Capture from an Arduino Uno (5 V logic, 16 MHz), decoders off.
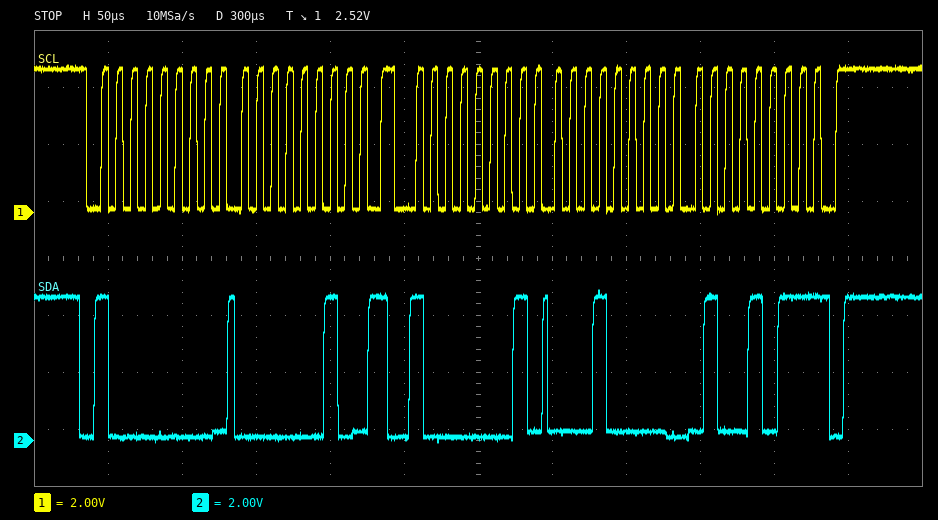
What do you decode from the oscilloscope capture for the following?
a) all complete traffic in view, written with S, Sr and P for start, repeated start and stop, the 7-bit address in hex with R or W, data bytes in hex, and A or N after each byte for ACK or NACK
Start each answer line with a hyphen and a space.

- S 40W A 02 A Sr 40R A 10 A 4B N P
